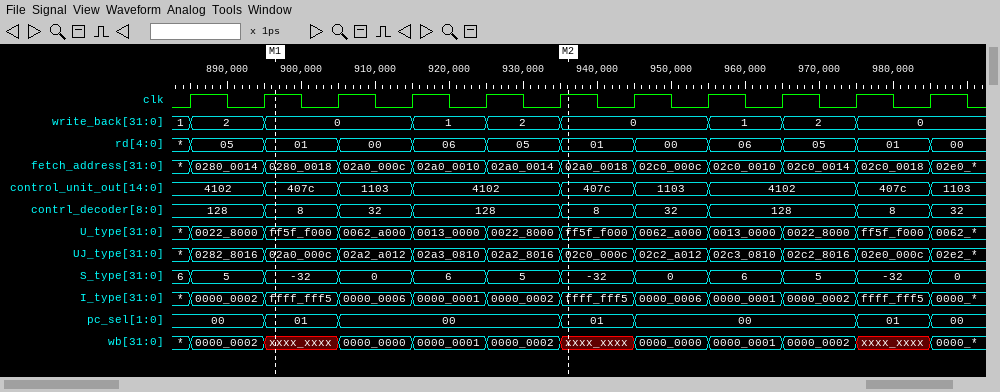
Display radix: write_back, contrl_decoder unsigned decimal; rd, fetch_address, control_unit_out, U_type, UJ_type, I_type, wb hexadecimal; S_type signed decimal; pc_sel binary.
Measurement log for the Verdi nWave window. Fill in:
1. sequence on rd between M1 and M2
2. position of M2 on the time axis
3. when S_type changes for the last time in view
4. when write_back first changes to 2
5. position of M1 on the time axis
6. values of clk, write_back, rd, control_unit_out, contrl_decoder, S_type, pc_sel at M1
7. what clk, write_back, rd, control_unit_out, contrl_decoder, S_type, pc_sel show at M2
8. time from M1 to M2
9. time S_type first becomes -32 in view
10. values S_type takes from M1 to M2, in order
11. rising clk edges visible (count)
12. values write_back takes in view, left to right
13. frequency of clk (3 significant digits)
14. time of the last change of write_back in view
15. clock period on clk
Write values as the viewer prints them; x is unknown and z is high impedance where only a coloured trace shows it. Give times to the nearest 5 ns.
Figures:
01, 00, 06, 05, 01
935 ns
985 ns
885 ns
895 ns
clk=1, write_back=0, rd=01, control_unit_out=407c, contrl_decoder=8, S_type=-32, pc_sel=01
clk=1, write_back=0, rd=01, control_unit_out=407c, contrl_decoder=8, S_type=-32, pc_sel=01
40 ns
895 ns
-32, 0, 6, 5, -32
11
1, 2, 0, 1, 2, 0, 1, 2, 0
100 MHz
975 ns
10 ns
